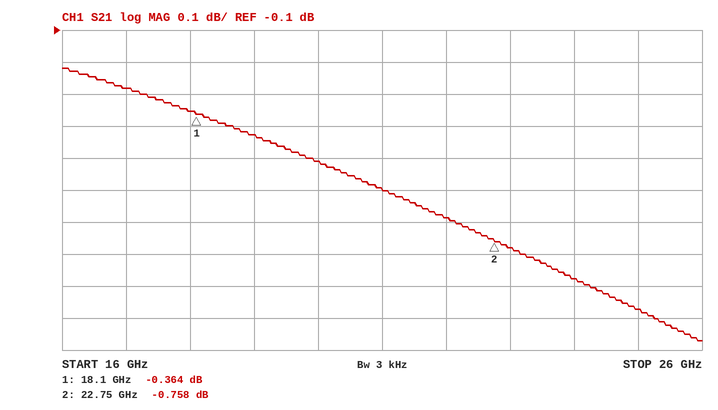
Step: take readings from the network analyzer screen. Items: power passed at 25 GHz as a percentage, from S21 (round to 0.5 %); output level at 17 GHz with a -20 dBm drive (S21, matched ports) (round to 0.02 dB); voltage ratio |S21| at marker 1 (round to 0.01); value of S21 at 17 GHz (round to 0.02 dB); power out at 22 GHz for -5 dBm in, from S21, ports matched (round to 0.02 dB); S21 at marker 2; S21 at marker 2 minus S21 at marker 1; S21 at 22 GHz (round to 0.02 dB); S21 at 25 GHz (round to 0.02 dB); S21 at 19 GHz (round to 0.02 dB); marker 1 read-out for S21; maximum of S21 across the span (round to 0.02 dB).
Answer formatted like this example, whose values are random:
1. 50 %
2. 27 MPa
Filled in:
1. 80.0 %
2. -20.28 dBm
3. 0.96
4. -0.28 dB
5. -5.68 dBm
6. -0.758 dB
7. -0.394 dB
8. -0.68 dB
9. -0.98 dB
10. -0.42 dB
11. -0.364 dB
12. -0.22 dB
